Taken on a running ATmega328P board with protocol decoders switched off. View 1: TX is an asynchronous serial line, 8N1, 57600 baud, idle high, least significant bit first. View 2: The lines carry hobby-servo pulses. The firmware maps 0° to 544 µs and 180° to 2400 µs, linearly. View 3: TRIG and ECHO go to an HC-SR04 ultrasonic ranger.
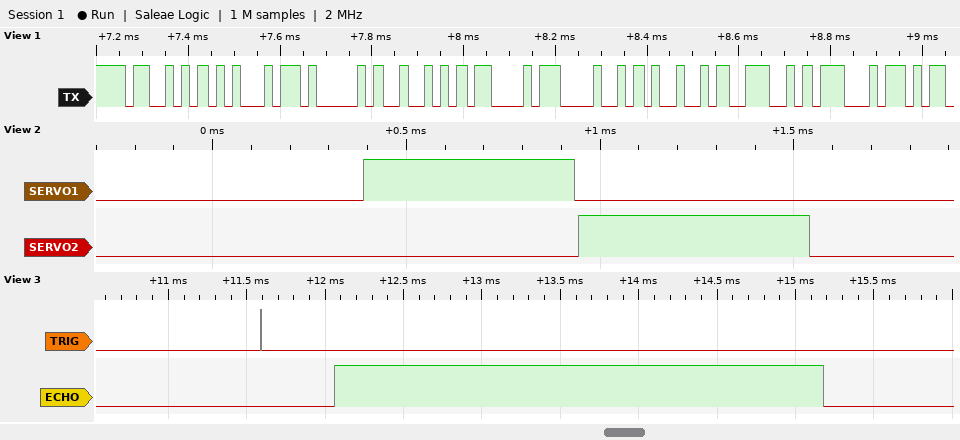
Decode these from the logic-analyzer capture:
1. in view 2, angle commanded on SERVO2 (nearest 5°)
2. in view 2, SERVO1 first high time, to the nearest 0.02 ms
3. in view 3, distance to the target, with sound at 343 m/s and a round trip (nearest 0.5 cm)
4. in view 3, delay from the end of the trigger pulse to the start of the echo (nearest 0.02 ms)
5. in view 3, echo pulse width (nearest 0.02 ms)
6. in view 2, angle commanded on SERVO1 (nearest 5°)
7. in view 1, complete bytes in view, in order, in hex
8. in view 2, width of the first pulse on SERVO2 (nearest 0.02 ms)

5°
0.54 ms
53.5 cm
0.46 ms
3.12 ms
0°
0x53 0x45 0x41 0x52 0x43 0x48 0x49 0x4E 0x47
0.60 ms
